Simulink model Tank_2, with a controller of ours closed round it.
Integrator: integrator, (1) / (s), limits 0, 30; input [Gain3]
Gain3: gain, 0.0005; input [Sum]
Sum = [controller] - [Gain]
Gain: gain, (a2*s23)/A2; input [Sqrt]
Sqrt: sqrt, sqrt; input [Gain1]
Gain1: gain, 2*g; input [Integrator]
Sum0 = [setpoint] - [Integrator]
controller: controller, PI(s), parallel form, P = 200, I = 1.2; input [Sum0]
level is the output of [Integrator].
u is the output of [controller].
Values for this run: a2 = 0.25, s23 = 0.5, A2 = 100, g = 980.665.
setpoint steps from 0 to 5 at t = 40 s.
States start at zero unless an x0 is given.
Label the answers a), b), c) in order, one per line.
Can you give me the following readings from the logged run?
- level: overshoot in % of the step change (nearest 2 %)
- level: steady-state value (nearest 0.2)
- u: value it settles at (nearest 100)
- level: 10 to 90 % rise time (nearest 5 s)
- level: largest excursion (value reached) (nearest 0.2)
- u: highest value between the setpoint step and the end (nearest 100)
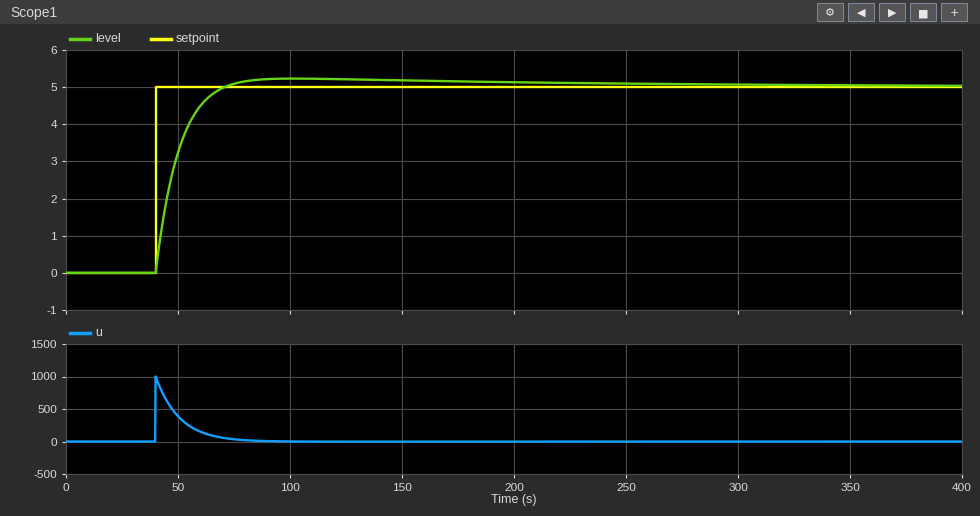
a) 4 %
b) 5.0
c) 0
d) 20 s
e) 5.2
f) 1000
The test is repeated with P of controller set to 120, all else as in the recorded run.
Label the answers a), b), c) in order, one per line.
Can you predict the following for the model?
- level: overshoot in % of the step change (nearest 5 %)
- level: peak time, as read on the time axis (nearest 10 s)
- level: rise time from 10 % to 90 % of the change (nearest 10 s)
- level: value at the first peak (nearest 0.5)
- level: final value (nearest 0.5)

a) 10 %
b) 120 s
c) 30 s
d) 5.5
e) 5.0
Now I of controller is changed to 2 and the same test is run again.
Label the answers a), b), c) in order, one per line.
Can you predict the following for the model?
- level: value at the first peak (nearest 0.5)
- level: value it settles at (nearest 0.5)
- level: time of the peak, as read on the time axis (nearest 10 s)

a) 5.5
b) 5.0
c) 90 s
